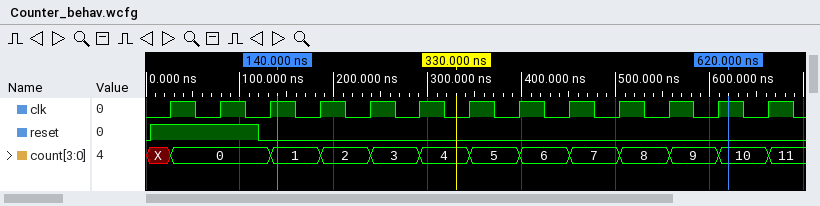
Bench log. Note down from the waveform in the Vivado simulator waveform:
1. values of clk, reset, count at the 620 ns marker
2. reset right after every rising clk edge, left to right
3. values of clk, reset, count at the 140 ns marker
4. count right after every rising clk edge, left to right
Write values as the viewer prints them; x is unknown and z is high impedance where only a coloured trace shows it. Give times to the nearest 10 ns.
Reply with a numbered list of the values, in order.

1. clk=1, reset=0, count=10
2. 1 1 0 0 0 0 0 0 0 0 0 0 0
3. clk=1, reset=0, count=1
4. 0, 0, 1, 2, 3, 4, 5, 6, 7, 8, 9, 10, 11
